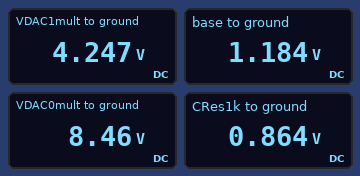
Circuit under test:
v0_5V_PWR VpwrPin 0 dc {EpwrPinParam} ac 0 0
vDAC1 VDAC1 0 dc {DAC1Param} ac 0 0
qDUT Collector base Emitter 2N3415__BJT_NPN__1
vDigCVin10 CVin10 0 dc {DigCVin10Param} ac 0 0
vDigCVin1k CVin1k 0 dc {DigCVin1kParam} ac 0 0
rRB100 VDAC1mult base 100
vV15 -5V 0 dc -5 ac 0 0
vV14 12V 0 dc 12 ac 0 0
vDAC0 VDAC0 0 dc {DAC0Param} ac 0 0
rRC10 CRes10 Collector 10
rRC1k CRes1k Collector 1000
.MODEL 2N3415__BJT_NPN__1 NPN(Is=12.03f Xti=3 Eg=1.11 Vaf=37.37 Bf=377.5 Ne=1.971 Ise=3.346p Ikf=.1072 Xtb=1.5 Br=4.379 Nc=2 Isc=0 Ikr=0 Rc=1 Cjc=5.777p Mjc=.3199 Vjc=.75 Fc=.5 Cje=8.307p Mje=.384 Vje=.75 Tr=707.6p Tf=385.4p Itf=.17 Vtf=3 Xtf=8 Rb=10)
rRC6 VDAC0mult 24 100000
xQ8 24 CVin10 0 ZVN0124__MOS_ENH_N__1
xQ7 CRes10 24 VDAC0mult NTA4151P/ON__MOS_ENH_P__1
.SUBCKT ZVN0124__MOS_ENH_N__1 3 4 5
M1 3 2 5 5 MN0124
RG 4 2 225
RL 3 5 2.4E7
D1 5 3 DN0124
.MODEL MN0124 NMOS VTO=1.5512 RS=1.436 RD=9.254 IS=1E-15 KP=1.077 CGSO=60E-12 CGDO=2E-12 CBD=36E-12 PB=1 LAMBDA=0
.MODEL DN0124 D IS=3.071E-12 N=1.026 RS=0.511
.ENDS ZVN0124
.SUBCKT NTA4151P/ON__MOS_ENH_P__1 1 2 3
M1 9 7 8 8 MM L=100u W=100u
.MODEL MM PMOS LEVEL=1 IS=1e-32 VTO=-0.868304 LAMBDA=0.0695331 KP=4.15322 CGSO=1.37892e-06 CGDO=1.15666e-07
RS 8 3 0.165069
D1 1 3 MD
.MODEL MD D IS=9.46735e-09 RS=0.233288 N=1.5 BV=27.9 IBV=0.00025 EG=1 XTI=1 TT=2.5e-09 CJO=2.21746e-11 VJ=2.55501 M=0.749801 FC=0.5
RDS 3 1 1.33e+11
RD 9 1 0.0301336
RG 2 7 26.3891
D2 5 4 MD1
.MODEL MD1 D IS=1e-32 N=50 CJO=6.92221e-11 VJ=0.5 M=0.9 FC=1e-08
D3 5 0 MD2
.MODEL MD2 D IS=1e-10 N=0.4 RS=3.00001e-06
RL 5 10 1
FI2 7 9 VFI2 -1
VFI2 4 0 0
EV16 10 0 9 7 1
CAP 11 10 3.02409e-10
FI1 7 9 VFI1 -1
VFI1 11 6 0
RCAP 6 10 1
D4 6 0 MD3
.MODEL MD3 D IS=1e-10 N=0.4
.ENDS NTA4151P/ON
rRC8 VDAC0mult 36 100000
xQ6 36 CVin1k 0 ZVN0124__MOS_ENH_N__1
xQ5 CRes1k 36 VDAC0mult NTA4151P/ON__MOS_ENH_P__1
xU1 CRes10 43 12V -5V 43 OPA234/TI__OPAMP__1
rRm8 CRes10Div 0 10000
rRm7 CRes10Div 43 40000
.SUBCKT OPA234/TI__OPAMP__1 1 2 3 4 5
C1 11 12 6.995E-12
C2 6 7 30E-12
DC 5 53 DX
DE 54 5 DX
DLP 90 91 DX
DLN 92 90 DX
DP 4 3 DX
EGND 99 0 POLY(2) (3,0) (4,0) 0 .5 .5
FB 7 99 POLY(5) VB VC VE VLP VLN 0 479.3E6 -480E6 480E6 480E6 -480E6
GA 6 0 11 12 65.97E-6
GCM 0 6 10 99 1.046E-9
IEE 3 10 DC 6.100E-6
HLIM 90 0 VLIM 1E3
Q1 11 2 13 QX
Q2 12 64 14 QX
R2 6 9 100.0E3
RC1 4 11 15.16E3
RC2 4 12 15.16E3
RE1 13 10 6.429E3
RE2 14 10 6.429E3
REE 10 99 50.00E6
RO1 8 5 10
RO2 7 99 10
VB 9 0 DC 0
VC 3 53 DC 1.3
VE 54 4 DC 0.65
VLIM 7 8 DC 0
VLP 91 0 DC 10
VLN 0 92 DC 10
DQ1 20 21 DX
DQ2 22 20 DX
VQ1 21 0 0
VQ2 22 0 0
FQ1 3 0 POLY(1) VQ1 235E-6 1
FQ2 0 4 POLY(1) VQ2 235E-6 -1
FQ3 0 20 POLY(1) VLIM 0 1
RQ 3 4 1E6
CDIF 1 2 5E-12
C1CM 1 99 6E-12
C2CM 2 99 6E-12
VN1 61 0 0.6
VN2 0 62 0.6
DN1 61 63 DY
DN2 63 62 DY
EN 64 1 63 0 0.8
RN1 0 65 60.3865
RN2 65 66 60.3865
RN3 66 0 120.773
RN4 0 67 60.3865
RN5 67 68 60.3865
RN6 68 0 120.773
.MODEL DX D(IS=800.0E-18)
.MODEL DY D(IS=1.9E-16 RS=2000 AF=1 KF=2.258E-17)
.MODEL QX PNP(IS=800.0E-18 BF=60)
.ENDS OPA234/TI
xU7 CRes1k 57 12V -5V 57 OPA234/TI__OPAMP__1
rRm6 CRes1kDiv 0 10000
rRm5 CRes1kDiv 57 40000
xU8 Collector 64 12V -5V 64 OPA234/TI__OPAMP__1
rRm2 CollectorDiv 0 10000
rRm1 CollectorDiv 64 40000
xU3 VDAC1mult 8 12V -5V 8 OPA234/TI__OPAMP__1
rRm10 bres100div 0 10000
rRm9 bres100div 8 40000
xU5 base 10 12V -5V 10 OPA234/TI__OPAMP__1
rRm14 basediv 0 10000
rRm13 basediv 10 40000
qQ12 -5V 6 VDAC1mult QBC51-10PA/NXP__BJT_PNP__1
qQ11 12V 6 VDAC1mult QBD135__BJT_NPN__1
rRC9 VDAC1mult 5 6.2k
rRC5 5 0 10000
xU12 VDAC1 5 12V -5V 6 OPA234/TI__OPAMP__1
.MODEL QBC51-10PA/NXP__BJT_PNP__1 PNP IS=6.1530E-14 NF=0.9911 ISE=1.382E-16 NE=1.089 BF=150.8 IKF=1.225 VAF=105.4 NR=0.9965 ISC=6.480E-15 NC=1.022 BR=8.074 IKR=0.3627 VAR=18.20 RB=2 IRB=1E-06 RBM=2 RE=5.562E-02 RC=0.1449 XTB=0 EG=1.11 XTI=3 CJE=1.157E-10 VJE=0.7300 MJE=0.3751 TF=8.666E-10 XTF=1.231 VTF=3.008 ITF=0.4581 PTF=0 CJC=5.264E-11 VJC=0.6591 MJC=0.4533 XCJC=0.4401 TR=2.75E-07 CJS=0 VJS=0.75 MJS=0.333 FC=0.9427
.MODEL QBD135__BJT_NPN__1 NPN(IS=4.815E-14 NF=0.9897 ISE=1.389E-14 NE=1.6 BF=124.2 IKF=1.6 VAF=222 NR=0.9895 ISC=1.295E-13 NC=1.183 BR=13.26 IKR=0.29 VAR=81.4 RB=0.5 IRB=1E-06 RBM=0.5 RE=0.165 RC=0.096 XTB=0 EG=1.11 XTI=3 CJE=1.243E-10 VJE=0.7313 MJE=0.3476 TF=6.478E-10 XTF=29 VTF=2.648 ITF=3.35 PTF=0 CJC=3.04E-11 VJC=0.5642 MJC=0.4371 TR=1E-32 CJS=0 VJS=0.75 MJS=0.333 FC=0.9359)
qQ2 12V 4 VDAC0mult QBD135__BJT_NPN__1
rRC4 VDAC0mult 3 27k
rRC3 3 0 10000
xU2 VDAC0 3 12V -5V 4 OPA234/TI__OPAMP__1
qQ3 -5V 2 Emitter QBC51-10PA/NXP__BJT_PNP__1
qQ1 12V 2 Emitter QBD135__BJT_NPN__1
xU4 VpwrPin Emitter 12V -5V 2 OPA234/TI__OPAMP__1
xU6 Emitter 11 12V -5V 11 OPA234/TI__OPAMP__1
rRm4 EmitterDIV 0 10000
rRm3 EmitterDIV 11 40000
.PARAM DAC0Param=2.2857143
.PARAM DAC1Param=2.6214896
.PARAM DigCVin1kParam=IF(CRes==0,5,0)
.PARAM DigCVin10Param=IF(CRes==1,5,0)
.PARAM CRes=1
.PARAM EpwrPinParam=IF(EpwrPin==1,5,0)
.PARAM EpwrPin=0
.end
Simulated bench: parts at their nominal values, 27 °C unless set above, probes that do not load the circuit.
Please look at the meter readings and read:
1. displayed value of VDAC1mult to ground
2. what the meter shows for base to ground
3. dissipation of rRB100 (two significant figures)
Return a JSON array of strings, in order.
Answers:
["4.247 V", "1.184 V", "94 mW"]
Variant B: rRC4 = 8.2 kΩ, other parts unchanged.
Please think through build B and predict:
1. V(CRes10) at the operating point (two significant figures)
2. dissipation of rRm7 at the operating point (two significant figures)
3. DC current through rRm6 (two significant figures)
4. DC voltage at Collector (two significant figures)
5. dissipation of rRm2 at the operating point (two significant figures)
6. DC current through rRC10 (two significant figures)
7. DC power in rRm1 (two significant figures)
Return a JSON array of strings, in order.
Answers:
["4.1 V", "260 µW", "8.8 µA", "440 mV", "770 nW", "360 mA", "3.1 µW"]
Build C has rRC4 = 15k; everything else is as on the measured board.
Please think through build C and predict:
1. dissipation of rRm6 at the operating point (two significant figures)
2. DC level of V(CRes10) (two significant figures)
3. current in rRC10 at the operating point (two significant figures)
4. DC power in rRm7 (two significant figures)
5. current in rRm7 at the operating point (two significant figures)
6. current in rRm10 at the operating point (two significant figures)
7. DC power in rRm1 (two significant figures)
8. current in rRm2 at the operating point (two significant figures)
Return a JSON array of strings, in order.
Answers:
["1.4 µW", "5.6 V", "500 mA", "500 µW", "110 µA", "85 µA", "5.6 µW", "12 µA"]
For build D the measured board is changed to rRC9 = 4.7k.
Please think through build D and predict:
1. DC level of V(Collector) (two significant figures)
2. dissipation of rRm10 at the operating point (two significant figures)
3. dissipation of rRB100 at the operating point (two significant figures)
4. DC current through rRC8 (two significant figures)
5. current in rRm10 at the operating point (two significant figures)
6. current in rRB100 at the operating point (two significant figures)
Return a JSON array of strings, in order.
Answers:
["870 mV", "59 µW", "73 mW", "350 nA", "77 µA", "27 mA"]
